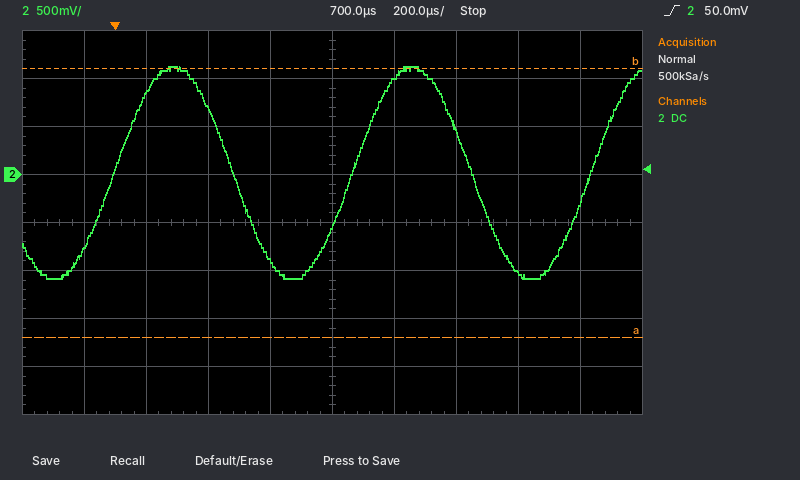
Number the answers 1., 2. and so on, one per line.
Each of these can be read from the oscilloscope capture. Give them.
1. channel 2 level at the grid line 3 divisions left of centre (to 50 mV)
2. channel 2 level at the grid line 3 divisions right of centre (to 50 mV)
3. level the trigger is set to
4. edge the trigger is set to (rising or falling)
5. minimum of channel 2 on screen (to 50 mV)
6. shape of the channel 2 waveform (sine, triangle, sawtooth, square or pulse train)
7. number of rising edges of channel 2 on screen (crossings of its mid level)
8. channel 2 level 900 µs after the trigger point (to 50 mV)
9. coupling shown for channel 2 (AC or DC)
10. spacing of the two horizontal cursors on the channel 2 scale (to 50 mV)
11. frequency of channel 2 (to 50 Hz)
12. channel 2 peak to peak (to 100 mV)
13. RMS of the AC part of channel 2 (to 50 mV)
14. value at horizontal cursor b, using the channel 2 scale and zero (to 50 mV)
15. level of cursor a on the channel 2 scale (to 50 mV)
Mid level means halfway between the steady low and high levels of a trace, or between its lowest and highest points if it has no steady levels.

1. 850 mV
2. -1.00 V
3. 50.0 mV
4. rising
5. -1.10 V
6. sine
7. 3
8. 1.00 V
9. DC
10. 2.80 V
11. 1.30 kHz
12. 2.20 V
13. 800 mV
14. 1.10 V
15. -1.70 V
